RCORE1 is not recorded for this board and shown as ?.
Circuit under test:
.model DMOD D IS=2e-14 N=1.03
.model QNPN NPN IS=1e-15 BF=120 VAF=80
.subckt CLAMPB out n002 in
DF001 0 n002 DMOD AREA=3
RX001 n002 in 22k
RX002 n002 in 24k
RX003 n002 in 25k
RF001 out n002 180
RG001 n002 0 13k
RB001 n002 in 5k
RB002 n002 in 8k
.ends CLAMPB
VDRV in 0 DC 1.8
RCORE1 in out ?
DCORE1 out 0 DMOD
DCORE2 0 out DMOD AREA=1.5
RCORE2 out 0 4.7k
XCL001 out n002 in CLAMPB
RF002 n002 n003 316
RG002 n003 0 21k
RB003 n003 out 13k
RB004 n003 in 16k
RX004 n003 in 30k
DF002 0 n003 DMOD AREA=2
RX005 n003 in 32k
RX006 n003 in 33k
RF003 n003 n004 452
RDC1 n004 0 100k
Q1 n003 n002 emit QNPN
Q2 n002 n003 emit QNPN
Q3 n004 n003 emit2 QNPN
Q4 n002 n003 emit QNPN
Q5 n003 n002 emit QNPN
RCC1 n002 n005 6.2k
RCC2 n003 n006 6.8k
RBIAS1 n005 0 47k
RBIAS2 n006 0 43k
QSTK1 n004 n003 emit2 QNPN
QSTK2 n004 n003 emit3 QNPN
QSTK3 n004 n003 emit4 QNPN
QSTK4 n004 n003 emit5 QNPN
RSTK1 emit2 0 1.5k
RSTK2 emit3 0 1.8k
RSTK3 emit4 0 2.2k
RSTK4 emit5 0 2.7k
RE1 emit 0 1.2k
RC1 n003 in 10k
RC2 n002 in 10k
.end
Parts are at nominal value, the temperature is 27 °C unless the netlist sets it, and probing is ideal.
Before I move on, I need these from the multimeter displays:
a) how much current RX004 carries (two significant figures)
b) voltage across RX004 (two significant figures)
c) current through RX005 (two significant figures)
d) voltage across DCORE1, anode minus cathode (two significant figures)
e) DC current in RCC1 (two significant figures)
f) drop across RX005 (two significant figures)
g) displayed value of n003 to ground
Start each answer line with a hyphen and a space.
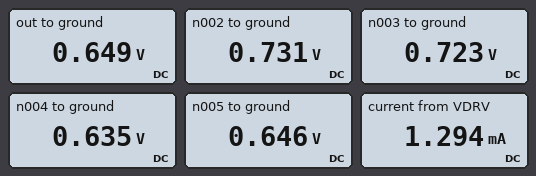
- 36 µA
- 1.1 V
- 34 µA
- 650 mV
- 14 µA
- 1.1 V
- 0.723 V
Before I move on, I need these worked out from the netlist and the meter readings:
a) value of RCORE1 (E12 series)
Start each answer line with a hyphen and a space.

- 2.7 kΩ
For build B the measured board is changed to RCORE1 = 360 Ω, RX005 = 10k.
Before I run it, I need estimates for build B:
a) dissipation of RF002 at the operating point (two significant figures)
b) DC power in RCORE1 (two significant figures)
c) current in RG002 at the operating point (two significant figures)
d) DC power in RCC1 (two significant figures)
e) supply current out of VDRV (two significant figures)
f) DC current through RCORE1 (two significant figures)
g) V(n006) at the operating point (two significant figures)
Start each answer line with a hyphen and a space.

- 300 nW
- 3.4 mW
- 36 µA
- 1.3 µW
- 4.0 mA
- 3.1 mA
- 650 mV
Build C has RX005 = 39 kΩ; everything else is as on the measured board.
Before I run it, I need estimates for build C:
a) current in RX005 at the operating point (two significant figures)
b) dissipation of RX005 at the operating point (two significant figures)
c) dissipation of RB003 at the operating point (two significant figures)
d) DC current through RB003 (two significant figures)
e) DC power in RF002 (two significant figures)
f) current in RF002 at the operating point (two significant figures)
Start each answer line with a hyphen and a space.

- 28 µA
- 30 µW
- 400 nW
- 5.6 µA
- 270 nW
- 29 µA
